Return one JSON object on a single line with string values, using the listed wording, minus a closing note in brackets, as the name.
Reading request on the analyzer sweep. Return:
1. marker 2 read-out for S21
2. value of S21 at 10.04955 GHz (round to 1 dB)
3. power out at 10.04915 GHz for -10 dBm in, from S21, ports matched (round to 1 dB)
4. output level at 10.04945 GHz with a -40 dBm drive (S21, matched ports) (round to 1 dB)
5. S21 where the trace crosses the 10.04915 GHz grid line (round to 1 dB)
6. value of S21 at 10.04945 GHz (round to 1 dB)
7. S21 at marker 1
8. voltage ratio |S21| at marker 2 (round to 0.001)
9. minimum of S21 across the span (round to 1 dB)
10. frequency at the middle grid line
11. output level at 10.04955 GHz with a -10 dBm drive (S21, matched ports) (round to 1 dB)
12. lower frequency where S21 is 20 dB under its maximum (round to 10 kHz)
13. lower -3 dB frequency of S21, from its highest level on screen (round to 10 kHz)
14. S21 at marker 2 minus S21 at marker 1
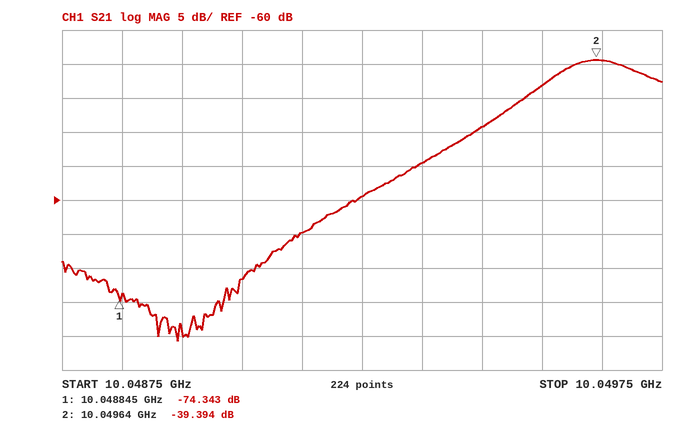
{"marker 2 read-out for S21": "-39.394 dB", "value of S21 at 10.04955 GHz": "-43 dB", "power out at 10.04915 GHz for -10 dBm in, from S21, ports matched": "-75 dBm", "output level at 10.04945 GHz with a -40 dBm drive (S21, matched ports)": "-89 dBm", "S21 where the trace crosses the 10.04915 GHz grid line": "-65 dB", "value of S21 at 10.04945 GHz": "-49 dB", "S21 at marker 1": "-74.343 dB", "voltage ratio |S21| at marker 2": "0.011", "minimum of S21 across the span": "-81 dB", "frequency at the middle grid line": "10.04925 GHz", "output level at 10.04955 GHz with a -10 dBm drive (S21, matched ports)": "-53 dBm", "lower frequency where S21 is 20 dB under its maximum": "10.04925 GHz", "lower -3 dB frequency of S21, from its highest level on screen": "10.04956 GHz", "S21 at marker 2 minus S21 at marker 1": "34.949 dB"}
